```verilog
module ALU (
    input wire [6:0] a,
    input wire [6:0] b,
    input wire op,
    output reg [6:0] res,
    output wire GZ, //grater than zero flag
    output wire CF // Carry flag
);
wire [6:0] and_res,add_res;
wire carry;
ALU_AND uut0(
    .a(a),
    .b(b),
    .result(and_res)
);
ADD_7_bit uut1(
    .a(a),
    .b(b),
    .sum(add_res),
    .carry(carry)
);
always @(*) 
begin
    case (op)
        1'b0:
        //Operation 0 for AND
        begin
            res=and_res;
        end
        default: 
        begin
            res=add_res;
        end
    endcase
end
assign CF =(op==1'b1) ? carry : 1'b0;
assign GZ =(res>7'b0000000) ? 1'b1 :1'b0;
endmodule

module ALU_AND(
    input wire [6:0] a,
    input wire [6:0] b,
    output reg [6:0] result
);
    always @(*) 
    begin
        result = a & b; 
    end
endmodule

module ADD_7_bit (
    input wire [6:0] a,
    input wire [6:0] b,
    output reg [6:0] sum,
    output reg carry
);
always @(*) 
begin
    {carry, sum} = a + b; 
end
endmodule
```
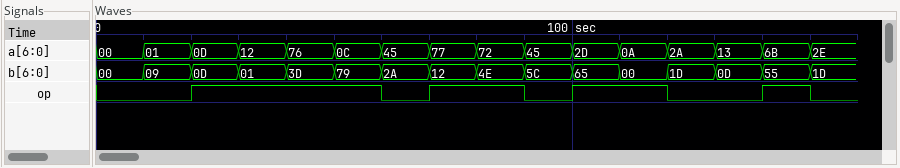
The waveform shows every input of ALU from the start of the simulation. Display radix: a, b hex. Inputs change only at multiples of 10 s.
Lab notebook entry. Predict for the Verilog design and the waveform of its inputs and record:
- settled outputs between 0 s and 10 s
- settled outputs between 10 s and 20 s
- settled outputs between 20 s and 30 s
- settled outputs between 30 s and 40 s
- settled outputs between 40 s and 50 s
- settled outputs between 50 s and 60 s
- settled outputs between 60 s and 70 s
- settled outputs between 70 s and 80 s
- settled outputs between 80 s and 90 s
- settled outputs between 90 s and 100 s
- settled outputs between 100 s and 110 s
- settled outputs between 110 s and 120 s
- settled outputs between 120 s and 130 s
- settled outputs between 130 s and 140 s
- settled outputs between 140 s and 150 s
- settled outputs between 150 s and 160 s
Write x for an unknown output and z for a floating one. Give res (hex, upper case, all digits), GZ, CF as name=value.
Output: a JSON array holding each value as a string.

["res=00, GZ=0, CF=0", "res=01, GZ=1, CF=0", "res=1A, GZ=1, CF=0", "res=13, GZ=1, CF=0", "res=33, GZ=1, CF=1", "res=05, GZ=1, CF=1", "res=00, GZ=0, CF=0", "res=09, GZ=1, CF=1", "res=40, GZ=1, CF=1", "res=44, GZ=1, CF=0", "res=12, GZ=1, CF=1", "res=0A, GZ=1, CF=0", "res=08, GZ=1, CF=0", "res=01, GZ=1, CF=0", "res=40, GZ=1, CF=1", "res=0C, GZ=1, CF=0"]
